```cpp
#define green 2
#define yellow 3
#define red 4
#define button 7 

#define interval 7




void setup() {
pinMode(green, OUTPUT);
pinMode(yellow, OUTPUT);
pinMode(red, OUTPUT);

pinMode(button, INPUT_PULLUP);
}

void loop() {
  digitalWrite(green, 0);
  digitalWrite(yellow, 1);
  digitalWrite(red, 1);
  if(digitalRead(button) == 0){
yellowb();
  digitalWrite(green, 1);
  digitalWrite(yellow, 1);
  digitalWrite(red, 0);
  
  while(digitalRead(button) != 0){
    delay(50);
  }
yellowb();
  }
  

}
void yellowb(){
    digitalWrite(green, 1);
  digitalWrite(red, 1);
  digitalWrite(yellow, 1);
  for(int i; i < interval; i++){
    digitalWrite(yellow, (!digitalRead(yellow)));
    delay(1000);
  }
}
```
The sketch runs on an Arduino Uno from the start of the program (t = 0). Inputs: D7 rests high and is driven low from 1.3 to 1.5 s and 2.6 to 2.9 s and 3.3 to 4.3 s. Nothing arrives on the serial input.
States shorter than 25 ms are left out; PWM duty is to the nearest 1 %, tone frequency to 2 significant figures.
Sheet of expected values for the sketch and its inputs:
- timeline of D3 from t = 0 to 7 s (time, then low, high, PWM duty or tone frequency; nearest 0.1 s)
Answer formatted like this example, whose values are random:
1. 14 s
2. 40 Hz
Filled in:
1. 0 s high; 1.3 s low; 2.3 s high; 3.3 s low; 4.3 s high; 5.3 s low; 6.3 s high
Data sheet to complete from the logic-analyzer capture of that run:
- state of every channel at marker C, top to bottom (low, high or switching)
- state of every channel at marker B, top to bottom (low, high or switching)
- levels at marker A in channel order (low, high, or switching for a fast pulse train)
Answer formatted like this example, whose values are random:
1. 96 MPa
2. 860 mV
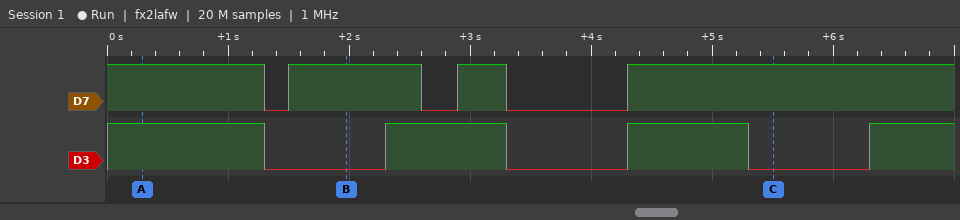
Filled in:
1. D7 high, D3 low
2. D7 high, D3 low
3. D7 high, D3 high
